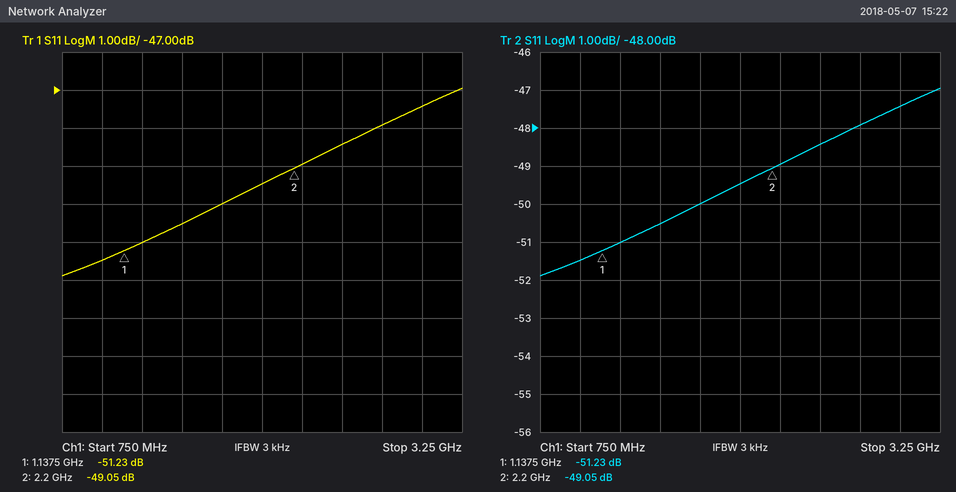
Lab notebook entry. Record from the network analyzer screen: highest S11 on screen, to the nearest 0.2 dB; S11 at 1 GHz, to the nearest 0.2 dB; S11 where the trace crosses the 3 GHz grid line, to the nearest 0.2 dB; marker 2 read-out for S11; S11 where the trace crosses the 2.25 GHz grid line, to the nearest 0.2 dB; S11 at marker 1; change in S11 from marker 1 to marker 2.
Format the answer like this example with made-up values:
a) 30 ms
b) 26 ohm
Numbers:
a) -47.0 dB
b) -51.4 dB
c) -47.4 dB
d) -49.05 dB
e) -49.0 dB
f) -51.23 dB
g) 2.18 dB
